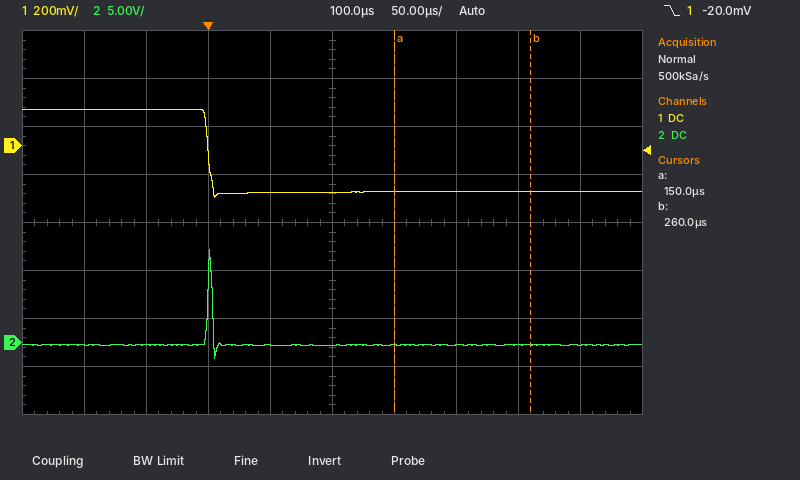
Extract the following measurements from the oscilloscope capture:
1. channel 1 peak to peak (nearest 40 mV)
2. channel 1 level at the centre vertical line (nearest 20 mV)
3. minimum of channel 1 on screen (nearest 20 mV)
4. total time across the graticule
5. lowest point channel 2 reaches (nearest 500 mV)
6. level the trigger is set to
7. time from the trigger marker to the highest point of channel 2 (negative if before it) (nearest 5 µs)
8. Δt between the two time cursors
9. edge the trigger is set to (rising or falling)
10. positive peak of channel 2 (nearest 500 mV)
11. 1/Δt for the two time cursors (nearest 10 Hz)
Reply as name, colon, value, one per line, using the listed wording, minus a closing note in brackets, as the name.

channel 1 peak to peak: 360 mV
channel 1 level at the centre vertical line: -200 mV
minimum of channel 1 on screen: -220 mV
total time across the graticule: 500 µs
lowest point channel 2 reaches: -1.5 V
level the trigger is set to: -20.0 mV
time from the trigger marker to the highest point of channel 2 (negative if before it): 0 µs
Δt between the two time cursors: 110 µs
edge the trigger is set to: falling
positive peak of channel 2: 9.5 V
1/Δt for the two time cursors: 9.09 kHz
